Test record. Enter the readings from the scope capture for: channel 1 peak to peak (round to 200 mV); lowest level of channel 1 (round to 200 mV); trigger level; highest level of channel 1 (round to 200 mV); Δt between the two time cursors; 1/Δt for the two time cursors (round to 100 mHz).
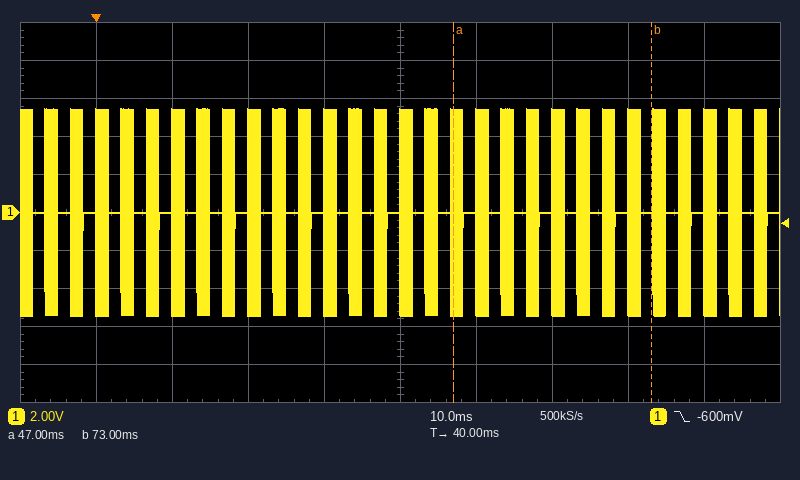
10.8 V
-5.4 V
-600 mV
5.4 V
26 ms
38.5 Hz
